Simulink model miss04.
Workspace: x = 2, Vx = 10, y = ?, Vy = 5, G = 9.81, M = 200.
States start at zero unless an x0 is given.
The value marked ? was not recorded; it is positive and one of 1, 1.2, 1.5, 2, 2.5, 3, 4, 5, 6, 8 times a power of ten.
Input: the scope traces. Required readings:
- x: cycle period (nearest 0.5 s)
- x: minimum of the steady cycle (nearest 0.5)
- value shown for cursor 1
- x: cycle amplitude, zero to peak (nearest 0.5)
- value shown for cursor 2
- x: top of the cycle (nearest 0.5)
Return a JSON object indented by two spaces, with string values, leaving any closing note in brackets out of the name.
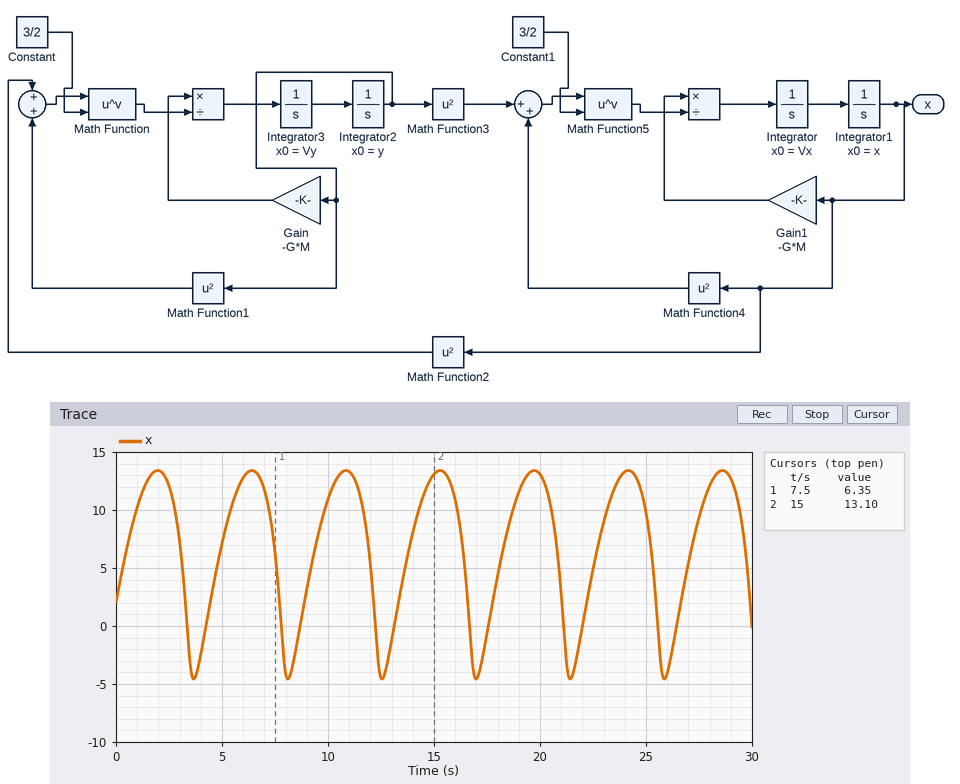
{
  "x: cycle period": "4.5 s",
  "x: minimum of the steady cycle": "-4.5",
  "value shown for cursor 1": "6.35",
  "x: cycle amplitude, zero to peak": "9.0",
  "value shown for cursor 2": "13.10",
  "x: top of the cycle": "13.5"
}
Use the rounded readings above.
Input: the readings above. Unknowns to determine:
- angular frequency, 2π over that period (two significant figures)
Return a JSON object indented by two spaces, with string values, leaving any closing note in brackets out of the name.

{
  "angular frequency, 2π over that period": "1.4 rad/s"
}
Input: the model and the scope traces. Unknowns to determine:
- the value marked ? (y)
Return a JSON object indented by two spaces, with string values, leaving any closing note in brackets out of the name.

{
  "the value marked ?": "12"
}
